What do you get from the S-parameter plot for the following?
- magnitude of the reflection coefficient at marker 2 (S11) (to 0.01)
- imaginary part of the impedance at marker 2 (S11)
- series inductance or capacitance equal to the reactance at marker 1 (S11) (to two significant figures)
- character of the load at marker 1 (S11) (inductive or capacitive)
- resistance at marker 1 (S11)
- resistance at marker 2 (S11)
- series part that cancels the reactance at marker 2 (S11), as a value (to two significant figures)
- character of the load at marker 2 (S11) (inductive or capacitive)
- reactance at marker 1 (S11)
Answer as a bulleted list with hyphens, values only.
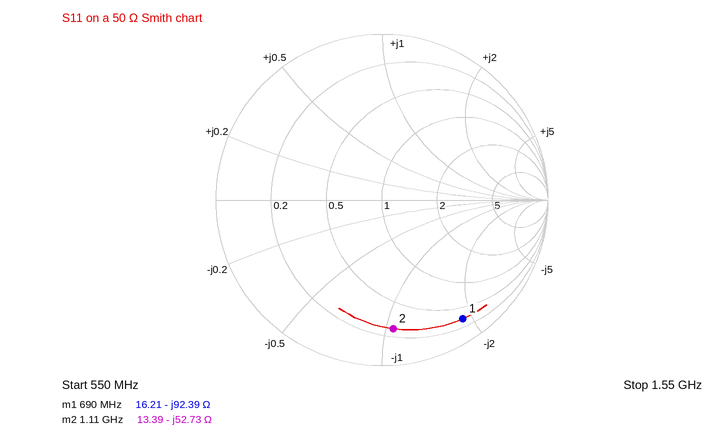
- 0.78
- -52.73 Ω
- 2.5 pF
- capacitive
- 16.21 Ω
- 13.39 Ω
- 7.6 nH
- capacitive
- -92.39 Ω
